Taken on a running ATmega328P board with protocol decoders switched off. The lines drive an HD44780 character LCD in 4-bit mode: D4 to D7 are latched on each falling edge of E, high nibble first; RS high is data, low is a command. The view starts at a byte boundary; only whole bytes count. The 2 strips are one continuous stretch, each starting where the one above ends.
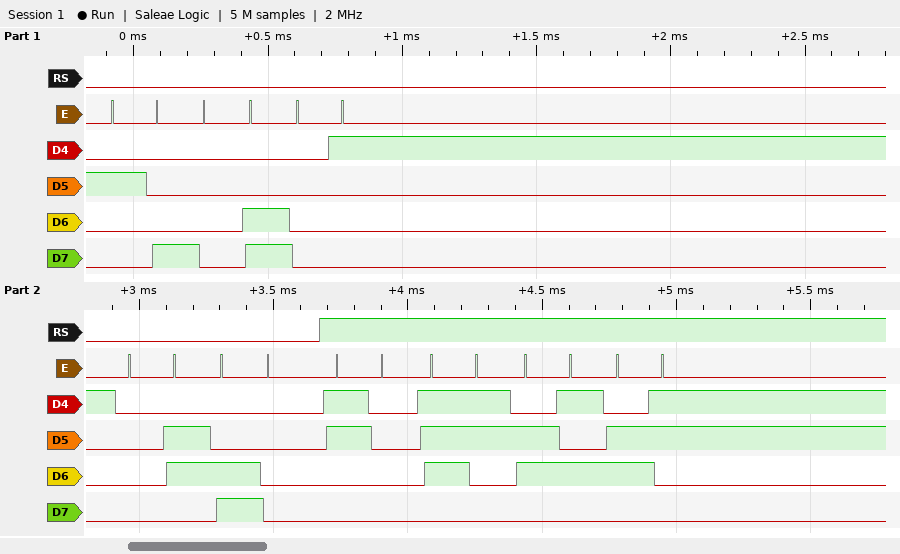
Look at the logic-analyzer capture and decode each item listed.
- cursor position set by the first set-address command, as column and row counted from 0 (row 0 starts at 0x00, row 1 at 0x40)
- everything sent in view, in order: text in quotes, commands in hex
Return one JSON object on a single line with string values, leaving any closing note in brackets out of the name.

{"cursor position set by the first set-address command, as column and row counted from 0": "column 0, row 1", "everything sent in view, in order: text in quotes, commands in hex": "0x28 0x0C 0x01 0x06 0xC0 \"0sec\""}
